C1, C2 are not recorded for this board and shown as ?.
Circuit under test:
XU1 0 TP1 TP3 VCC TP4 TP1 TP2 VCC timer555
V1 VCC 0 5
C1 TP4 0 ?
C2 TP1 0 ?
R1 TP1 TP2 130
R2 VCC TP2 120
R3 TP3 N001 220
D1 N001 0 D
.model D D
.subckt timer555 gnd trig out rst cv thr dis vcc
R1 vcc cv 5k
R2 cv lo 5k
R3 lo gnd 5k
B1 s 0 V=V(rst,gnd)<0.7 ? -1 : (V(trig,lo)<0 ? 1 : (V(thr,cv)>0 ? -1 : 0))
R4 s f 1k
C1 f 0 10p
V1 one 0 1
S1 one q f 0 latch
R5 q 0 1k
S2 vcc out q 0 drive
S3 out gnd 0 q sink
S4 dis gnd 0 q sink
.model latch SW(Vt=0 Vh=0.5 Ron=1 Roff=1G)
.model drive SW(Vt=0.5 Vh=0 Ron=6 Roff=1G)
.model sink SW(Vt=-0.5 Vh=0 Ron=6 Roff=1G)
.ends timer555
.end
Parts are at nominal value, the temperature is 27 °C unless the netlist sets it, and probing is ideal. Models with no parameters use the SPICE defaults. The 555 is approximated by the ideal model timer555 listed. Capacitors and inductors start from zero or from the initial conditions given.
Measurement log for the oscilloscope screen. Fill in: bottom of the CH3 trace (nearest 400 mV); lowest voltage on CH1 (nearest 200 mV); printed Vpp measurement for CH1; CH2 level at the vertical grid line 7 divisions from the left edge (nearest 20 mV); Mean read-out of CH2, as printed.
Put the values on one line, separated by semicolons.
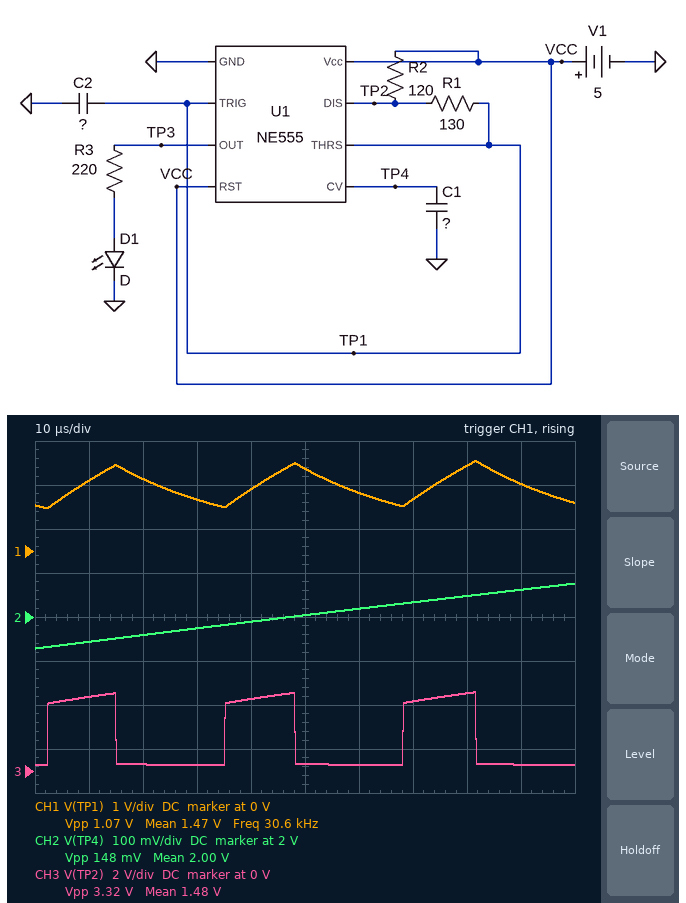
400 mV; 1.0 V; 1.07 V; 2.04 V; 2.00 V
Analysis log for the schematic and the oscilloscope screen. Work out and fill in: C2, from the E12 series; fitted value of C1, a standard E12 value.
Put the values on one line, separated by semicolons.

180 nF; 270 nF
